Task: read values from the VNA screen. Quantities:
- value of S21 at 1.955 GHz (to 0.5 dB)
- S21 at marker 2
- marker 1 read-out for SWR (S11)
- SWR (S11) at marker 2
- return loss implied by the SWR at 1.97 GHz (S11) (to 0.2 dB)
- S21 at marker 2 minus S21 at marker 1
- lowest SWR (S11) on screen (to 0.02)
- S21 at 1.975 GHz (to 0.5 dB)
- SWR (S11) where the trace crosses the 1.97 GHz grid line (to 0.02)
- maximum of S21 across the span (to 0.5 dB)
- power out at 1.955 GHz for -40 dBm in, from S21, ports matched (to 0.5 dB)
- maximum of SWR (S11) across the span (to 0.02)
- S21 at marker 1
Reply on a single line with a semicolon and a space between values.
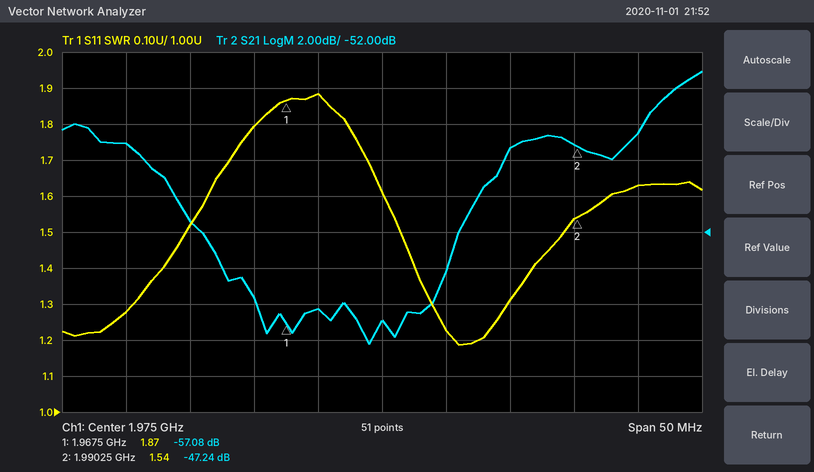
-47.0 dB; -47.24 dB; 1.87; 1.54; 10.2 dB; 9.84 dB; 1.18; -57.0 dB; 1.88; -43.0 dB; -87.0 dBm; 1.88; -57.08 dB
